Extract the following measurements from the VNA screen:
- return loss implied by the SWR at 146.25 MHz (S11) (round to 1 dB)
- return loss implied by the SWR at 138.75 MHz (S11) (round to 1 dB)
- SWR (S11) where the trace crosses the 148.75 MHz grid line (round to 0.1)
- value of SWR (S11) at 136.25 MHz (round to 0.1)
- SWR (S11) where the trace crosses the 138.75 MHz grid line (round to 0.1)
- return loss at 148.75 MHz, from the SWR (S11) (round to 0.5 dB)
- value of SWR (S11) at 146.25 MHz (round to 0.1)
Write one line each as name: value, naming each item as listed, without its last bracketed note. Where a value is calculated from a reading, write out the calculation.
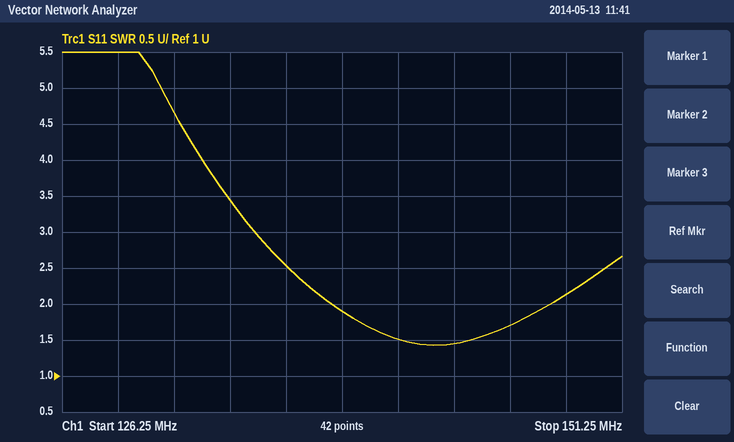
return loss implied by the SWR at 146.25 MHz (S11): −20 log10((1.7 − 1)/(1.7 + 1)) ≈ 12 dB
return loss implied by the SWR at 138.75 MHz (S11): −20 log10((1.9 − 1)/(1.9 + 1)) ≈ 10 dB
SWR (S11) where the trace crosses the 148.75 MHz grid line: 2.1
value of SWR (S11) at 136.25 MHz: 2.5
SWR (S11) where the trace crosses the 138.75 MHz grid line: 1.9
return loss at 148.75 MHz, from the SWR (S11): −20 log10((2.1 − 1)/(2.1 + 1)) ≈ 9.0 dB
value of SWR (S11) at 146.25 MHz: 1.7
